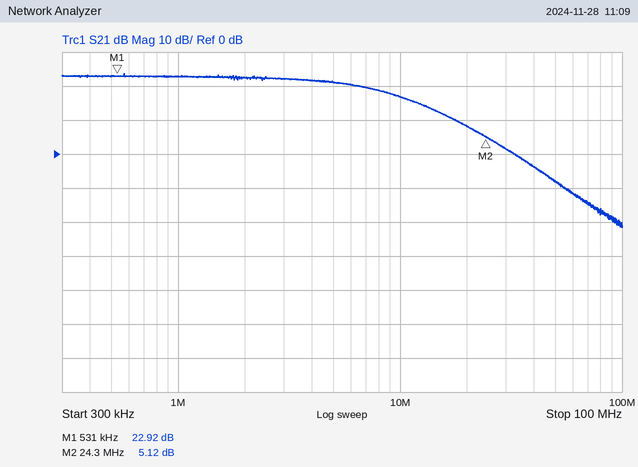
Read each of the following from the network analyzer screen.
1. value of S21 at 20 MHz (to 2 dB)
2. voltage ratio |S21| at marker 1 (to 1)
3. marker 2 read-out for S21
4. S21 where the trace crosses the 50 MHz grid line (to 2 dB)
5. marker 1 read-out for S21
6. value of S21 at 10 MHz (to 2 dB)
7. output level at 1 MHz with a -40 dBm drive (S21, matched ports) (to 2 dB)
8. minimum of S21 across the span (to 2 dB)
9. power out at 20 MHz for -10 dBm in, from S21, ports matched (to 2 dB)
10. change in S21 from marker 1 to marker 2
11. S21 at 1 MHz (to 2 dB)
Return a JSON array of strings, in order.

["8 dB", "14", "5.12 dB", "-8 dB", "22.92 dB", "16 dB", "-18 dBm", "-22 dB", "-2 dBm", "-17.80 dB", "22 dB"]
